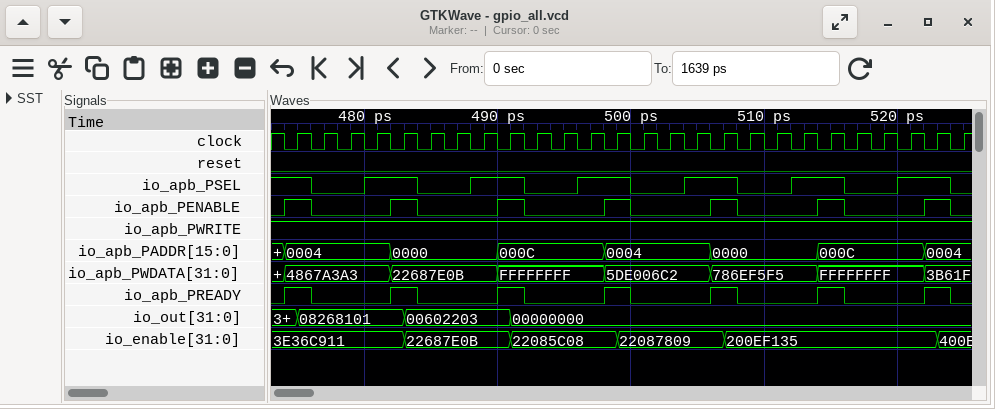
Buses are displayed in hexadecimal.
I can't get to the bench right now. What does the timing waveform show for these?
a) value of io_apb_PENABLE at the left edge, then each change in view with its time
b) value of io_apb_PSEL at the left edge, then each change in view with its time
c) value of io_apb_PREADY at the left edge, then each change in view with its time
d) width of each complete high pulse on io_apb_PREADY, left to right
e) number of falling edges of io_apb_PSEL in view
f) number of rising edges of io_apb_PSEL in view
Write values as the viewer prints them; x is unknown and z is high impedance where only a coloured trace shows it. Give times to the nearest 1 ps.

0, 1 at 474 ps, 0 at 476 ps, 1 at 482 ps, 0 at 484 ps, 1 at 490 ps, 0 at 492 ps, 1 at 498 ps, 0 at 500 ps, 1 at 506 ps, 0 at 508 ps, 1 at 514 ps, 0 at 516 ps, 1 at 522 ps, 0 at 524 ps
1, 0 at 476 ps, 1 at 480 ps, 0 at 484 ps, 1 at 488 ps, 0 at 492 ps, 1 at 496 ps, 0 at 500 ps, 1 at 504 ps, 0 at 508 ps, 1 at 512 ps, 0 at 516 ps, 1 at 520 ps, 0 at 524 ps
0, 1 at 474 ps, 0 at 476 ps, 1 at 482 ps, 0 at 484 ps, 1 at 490 ps, 0 at 492 ps, 1 at 498 ps, 0 at 500 ps, 1 at 506 ps, 0 at 508 ps, 1 at 514 ps, 0 at 516 ps, 1 at 522 ps, 0 at 524 ps
2 ps, 2 ps, 2 ps, 2 ps, 2 ps, 2 ps, 2 ps
7
6
